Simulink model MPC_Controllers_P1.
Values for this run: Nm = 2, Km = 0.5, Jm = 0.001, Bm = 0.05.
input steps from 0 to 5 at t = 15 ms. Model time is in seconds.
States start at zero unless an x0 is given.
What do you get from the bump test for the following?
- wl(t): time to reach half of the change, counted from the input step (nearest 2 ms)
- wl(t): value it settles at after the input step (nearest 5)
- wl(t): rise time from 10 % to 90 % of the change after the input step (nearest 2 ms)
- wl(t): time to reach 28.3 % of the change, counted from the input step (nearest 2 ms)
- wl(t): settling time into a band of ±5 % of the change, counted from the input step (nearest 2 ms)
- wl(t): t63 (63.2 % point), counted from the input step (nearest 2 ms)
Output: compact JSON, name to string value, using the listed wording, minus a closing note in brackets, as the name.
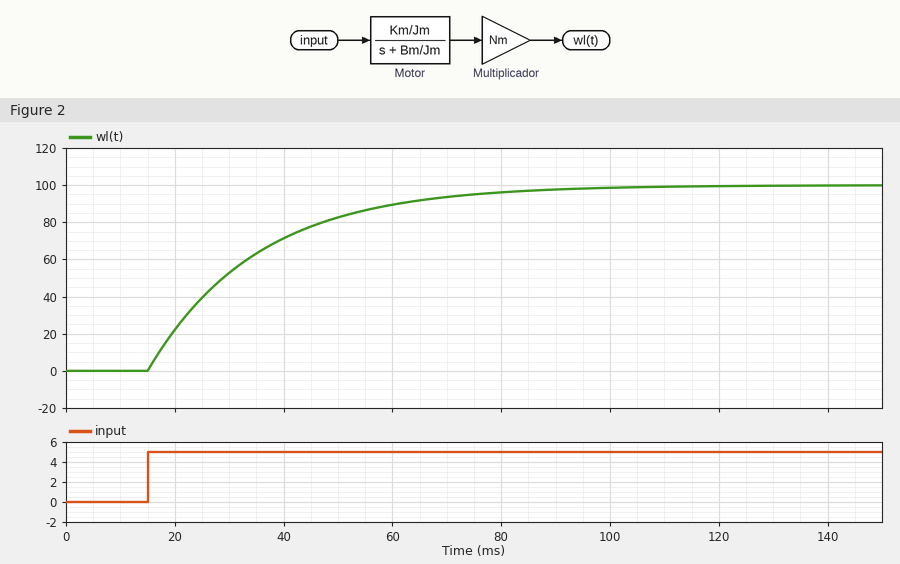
{"wl(t): time to reach half of the change, counted from the input step": "14 ms", "wl(t): value it settles at after the input step": "100", "wl(t): rise time from 10 % to 90 % of the change after the input step": "44 ms", "wl(t): time to reach 28.3 % of the change, counted from the input step": "6 ms", "wl(t): settling time into a band of ±5 % of the change, counted from the input step": "60 ms", "wl(t): t63 (63.2 % point), counted from the input step": "20 ms"}
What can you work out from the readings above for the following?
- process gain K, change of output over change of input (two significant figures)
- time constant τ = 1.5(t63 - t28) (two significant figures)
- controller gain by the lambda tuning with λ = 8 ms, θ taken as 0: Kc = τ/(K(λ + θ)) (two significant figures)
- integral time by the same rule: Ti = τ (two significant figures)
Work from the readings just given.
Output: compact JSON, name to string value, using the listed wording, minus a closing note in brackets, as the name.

{"process gain K, change of output over change of input": "20", "time constant τ = 1.5(t63 - t28)": "21 ms", "controller gain by the lambda tuning with λ = 8 ms, θ taken as 0: Kc = τ/(K(λ + θ))": "0.13", "integral time by the same rule: Ti = τ": "21 ms"}
